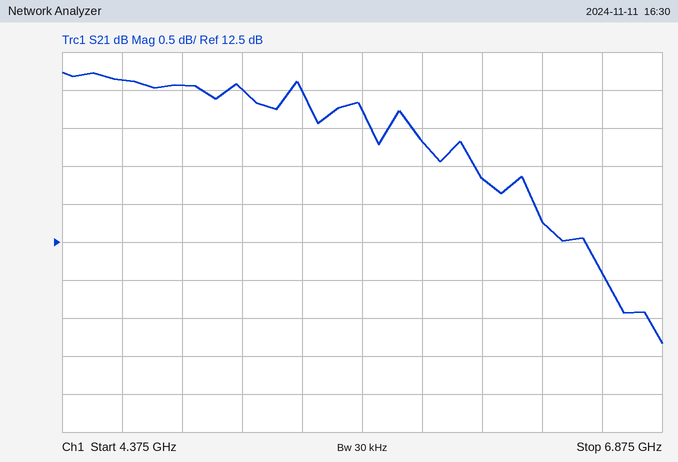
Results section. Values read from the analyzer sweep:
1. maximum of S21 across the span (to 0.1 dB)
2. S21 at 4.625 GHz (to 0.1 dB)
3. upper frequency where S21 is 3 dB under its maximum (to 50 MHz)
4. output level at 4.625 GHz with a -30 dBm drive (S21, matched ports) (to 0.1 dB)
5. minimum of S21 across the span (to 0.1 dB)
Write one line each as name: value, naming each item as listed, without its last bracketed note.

maximum of S21 across the span: 14.7 dB
S21 at 4.625 GHz: 14.6 dB
upper frequency where S21 is 3 dB under its maximum: 6.70 GHz
output level at 4.625 GHz with a -30 dBm drive (S21, matched ports): -15.4 dBm
minimum of S21 across the span: 11.2 dB
